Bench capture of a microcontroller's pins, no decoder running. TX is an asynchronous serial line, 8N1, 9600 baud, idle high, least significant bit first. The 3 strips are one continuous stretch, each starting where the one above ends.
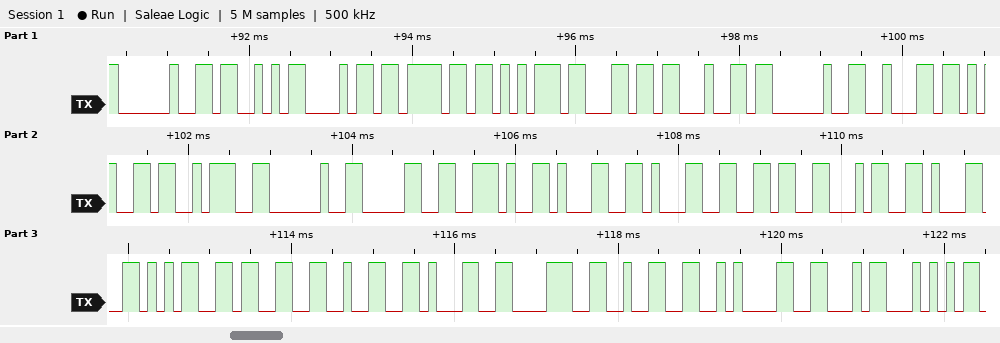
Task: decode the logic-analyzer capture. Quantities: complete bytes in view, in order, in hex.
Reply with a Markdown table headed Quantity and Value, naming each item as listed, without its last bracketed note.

| Quantity | Value |
|---|---|
| complete bytes in view, in order, in hex | 0x20 0x53 0x68 0x6F 0x75 0x6C 0x64 0x20 0x62 0x65 0x3A 0x20 0x30 0x2E 0x31 0x31 0x36 0x34 0x31 0x35 0x33 0x32 0x31 0x38 0x32 0x0A 0x46 0x54 |
